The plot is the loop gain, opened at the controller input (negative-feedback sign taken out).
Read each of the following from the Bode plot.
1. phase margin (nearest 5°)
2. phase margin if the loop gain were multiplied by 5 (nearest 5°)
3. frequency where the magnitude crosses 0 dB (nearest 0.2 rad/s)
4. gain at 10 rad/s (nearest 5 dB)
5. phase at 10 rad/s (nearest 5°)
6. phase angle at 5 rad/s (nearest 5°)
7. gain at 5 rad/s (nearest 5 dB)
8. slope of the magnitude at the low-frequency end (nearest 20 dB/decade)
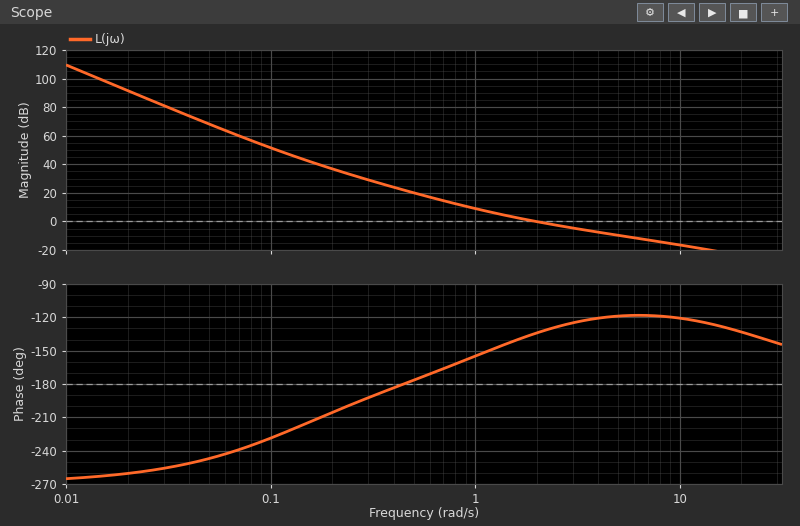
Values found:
45°
60°
2.0 rad/s
-15 dB
-120°
-120°
-10 dB
-60 dB/decade
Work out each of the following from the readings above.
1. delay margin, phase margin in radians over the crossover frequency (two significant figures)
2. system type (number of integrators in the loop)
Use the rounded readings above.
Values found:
0.39 s
3
